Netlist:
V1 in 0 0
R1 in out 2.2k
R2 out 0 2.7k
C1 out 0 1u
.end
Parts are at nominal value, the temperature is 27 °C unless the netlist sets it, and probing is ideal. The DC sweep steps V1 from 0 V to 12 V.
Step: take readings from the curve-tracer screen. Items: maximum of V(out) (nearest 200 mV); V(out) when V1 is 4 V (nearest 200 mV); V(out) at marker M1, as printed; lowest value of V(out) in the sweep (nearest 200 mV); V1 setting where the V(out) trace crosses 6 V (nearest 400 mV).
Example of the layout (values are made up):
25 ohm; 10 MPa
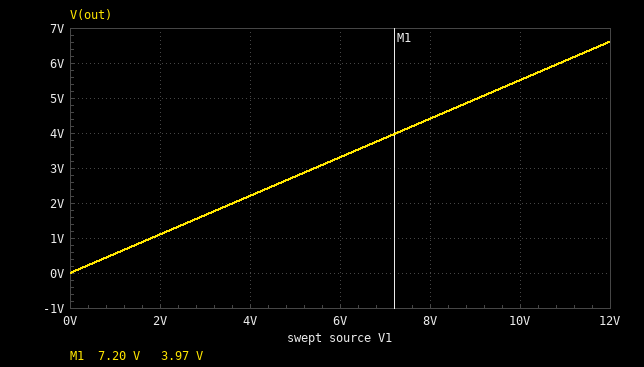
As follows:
6.6 V; 2.2 V; 3.97 V; 0 V; 10.8 V
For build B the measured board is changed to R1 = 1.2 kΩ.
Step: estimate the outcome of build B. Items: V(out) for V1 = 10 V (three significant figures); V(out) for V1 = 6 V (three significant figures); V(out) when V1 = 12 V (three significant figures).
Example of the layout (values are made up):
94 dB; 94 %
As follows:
6.92 V; 4.15 V; 8.31 V
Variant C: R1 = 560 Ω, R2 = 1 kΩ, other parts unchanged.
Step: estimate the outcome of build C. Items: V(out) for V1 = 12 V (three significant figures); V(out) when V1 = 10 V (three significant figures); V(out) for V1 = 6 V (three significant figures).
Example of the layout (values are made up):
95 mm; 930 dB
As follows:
7.69 V; 6.41 V; 3.85 V
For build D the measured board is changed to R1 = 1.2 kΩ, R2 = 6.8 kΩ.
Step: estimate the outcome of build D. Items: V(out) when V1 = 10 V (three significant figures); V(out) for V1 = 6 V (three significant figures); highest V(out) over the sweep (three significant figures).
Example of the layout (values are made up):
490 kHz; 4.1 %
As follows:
8.50 V; 5.10 V; 10.2 V
